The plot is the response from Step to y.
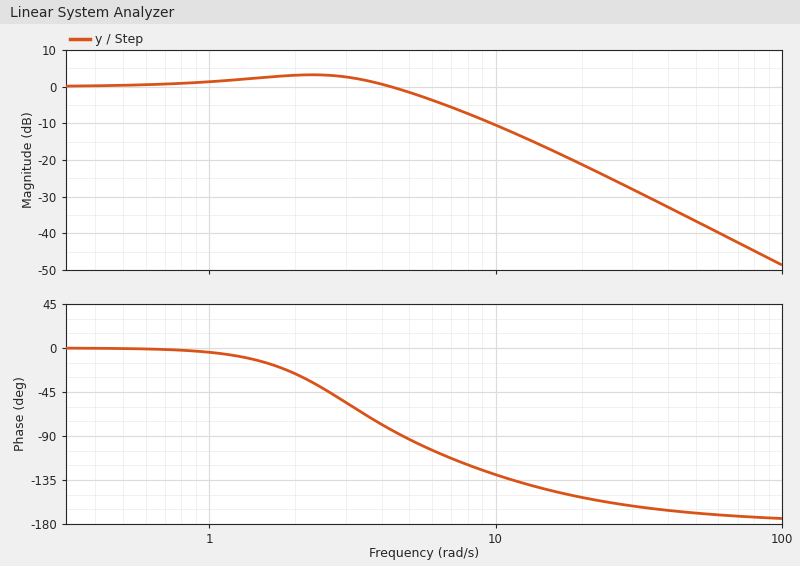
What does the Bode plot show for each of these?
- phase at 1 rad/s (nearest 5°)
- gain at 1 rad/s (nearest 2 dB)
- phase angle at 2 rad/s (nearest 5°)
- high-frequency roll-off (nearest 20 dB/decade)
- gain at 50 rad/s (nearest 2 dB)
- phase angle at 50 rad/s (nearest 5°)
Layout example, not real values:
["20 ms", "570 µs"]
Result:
["-5°", "2 dB", "-25°", "-40 dB/decade", "-36 dB", "-170°"]
